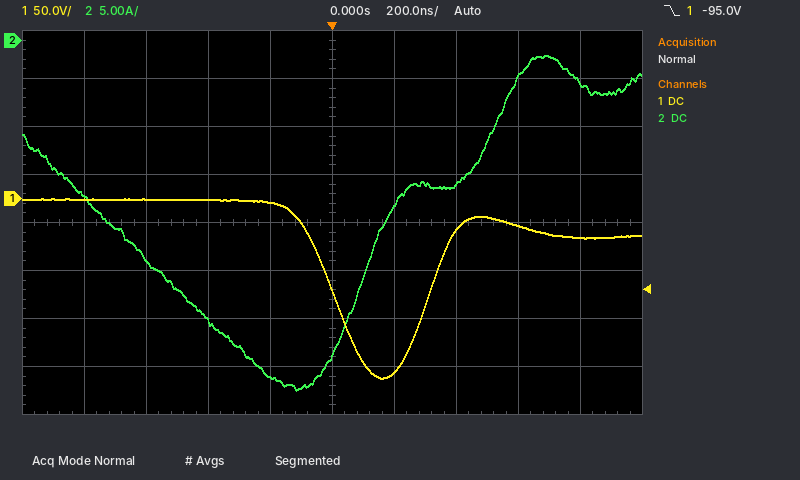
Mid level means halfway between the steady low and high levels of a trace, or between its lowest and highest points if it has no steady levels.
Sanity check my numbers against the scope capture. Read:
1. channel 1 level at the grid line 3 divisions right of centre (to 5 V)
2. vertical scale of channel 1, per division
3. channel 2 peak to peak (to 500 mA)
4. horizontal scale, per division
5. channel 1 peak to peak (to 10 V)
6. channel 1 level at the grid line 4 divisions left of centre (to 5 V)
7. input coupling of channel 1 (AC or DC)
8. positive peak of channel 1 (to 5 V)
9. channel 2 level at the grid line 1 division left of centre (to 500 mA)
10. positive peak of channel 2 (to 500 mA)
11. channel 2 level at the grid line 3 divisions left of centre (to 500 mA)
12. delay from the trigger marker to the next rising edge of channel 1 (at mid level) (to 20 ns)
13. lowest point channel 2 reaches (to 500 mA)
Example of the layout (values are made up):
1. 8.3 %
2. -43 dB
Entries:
1. -30 V
2. 50 V
3. 35.0 A
4. 200 ns
5. 190 V
6. 0 V
7. DC
8. 0 V
9. -35.0 A
10. -1.5 A
11. -23.0 A
12. 320 ns
13. -36.5 A
